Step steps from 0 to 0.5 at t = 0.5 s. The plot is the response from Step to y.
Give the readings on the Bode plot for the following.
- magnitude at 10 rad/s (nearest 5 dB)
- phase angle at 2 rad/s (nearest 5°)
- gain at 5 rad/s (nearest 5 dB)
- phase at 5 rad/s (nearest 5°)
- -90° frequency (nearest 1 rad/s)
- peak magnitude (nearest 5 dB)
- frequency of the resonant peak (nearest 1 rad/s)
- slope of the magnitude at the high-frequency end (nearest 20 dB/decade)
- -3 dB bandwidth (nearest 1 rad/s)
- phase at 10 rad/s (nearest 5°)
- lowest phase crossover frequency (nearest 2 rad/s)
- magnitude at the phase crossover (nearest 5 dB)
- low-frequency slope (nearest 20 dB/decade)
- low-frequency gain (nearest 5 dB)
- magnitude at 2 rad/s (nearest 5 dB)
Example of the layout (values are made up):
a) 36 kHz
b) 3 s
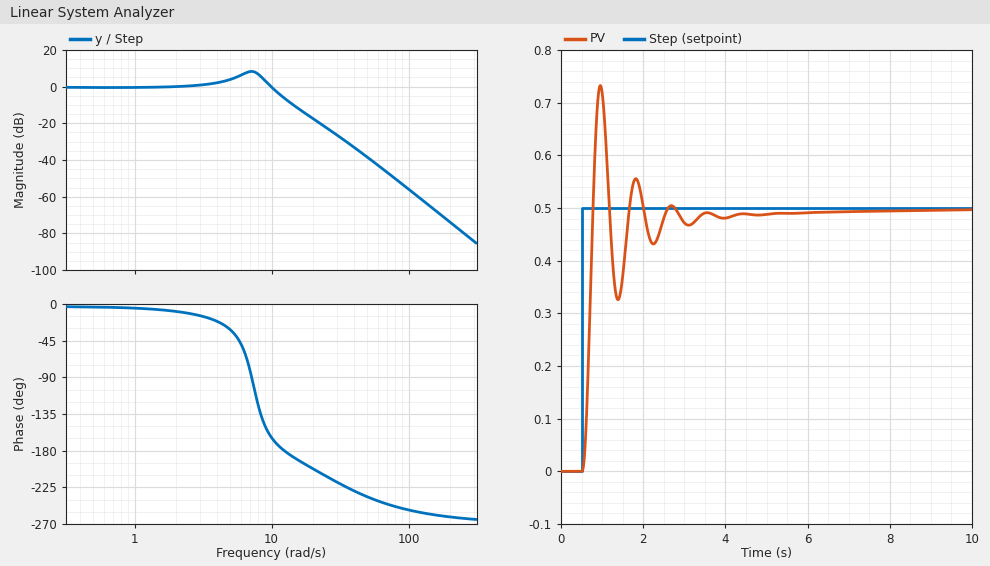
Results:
a) 0 dB
b) -10°
c) 5 dB
d) -30°
e) 7 rad/s
f) 10 dB
g) 7 rad/s
h) -60 dB/decade
i) 11 rad/s
j) -165°
k) 12 rad/s
l) -5 dB
m) 0 dB/decade
n) 0 dB
o) 0 dB
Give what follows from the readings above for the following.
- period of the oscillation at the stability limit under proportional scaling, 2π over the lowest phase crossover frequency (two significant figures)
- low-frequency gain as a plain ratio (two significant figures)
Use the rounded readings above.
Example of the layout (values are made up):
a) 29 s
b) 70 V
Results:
a) 0.52 s
b) 1.0
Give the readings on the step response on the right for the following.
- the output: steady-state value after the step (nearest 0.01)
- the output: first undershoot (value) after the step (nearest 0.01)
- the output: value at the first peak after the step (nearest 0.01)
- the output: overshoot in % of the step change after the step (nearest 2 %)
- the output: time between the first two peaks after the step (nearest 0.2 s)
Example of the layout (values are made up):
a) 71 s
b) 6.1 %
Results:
a) 0.50
b) 0.33
c) 0.73
d) 46 %
e) 0.8 s
